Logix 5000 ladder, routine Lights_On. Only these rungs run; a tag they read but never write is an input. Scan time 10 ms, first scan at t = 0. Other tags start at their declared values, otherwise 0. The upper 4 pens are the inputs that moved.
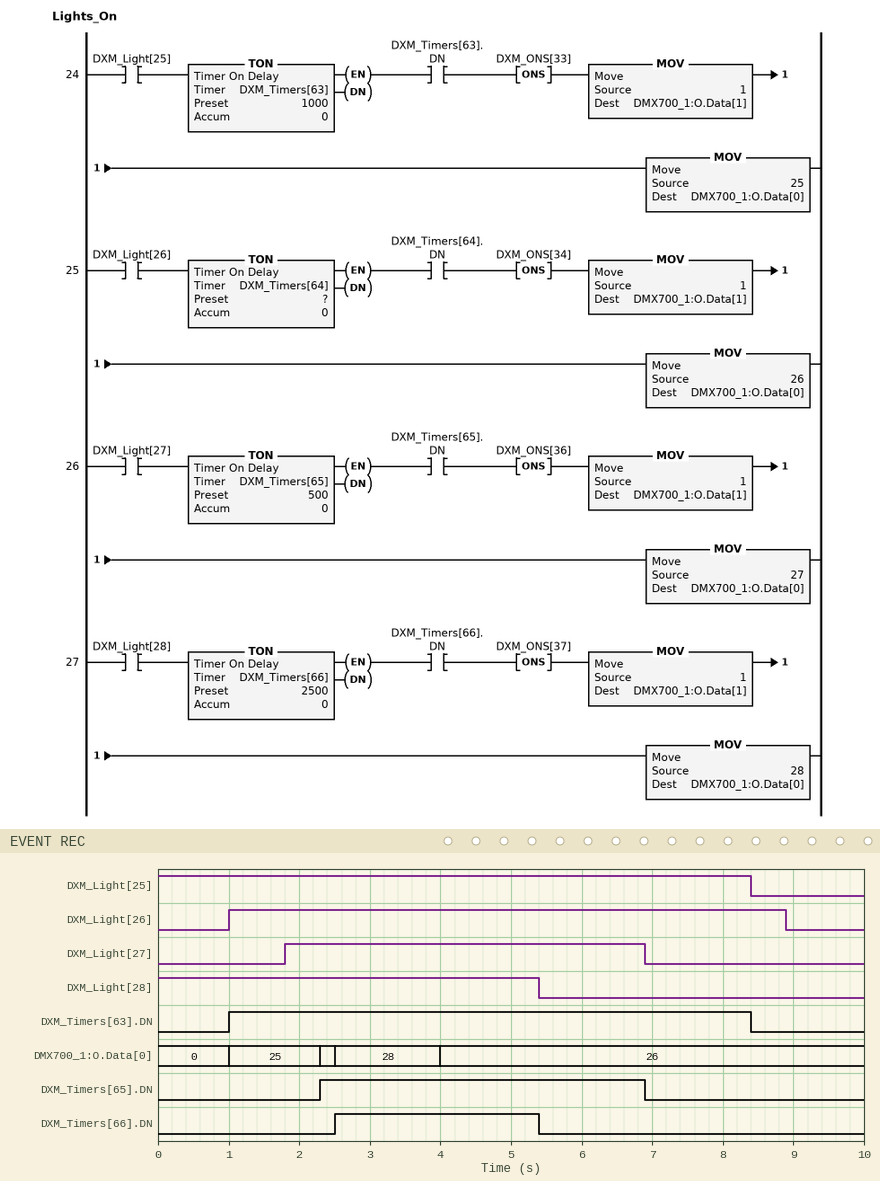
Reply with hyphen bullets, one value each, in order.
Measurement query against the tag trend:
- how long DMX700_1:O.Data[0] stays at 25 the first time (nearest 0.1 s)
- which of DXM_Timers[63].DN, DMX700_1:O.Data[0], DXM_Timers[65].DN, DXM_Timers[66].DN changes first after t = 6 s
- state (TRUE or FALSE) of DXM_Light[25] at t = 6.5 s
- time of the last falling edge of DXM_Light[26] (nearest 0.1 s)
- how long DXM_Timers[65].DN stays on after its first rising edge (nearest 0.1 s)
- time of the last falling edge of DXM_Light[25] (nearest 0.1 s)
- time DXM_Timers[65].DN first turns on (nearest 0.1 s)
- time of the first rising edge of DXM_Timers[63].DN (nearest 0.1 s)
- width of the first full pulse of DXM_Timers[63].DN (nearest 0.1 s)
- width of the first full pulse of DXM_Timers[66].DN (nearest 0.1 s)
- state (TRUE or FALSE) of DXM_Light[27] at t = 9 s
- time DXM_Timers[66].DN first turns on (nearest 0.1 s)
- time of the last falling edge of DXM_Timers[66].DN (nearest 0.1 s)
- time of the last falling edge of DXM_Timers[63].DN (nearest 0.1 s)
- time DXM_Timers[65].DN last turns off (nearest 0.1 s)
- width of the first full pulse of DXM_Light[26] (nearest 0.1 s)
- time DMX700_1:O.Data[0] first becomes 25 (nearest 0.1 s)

- 1.3 s
- DXM_Timers[65].DN
- TRUE
- 8.9 s
- 4.6 s
- 8.4 s
- 2.3 s
- 1.0 s
- 7.4 s
- 2.9 s
- FALSE
- 2.5 s
- 5.4 s
- 8.4 s
- 6.9 s
- 7.9 s
- 1.0 s
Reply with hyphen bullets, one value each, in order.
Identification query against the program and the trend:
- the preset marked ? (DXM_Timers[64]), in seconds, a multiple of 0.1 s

- 3.0 s
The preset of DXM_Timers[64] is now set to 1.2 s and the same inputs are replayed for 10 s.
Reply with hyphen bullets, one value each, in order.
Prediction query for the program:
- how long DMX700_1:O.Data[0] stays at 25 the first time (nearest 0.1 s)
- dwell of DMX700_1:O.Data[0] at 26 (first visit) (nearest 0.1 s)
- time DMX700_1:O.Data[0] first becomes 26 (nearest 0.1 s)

- 1.2 s
- 0.1 s
- 2.2 s
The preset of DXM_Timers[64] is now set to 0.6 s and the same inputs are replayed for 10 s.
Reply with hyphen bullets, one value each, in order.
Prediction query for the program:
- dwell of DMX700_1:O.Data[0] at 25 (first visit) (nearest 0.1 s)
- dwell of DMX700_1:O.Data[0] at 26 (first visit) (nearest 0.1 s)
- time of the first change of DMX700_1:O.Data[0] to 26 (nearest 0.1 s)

- 0.6 s
- 0.7 s
- 1.6 s
